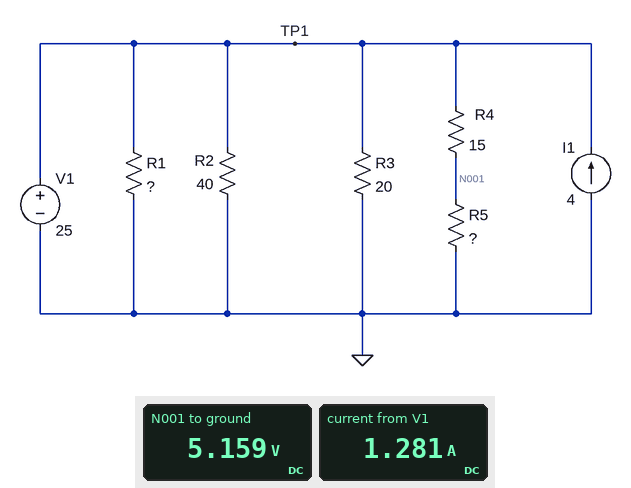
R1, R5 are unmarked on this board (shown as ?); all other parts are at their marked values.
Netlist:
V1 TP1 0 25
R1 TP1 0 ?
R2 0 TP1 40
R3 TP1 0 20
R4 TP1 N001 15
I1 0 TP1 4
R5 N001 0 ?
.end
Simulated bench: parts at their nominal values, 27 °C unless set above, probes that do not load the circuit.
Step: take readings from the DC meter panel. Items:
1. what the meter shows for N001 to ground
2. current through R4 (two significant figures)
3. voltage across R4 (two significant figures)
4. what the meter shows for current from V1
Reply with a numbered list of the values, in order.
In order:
1. 5.159 V
2. 1.3 A
3. 20 V
4. 1.281 A
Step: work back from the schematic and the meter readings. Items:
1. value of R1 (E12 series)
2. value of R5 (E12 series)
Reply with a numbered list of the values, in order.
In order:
1. 12 Ω
2. 3.9 Ω
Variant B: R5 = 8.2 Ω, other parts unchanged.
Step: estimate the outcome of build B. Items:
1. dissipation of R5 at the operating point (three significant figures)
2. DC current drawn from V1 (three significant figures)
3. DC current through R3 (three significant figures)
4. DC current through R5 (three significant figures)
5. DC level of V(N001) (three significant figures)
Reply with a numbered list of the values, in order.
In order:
1. 9.52 W
2. 1.04 A
3. 1.25 A
4. 1.08 A
5. 8.84 V
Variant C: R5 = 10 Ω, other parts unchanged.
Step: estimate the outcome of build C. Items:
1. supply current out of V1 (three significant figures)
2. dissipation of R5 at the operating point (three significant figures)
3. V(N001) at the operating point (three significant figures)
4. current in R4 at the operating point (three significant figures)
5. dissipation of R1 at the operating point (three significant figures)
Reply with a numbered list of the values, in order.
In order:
1. 958 mA
2. 10.0 W
3. 10.0 V
4. 1.00 A
5. 52.1 W
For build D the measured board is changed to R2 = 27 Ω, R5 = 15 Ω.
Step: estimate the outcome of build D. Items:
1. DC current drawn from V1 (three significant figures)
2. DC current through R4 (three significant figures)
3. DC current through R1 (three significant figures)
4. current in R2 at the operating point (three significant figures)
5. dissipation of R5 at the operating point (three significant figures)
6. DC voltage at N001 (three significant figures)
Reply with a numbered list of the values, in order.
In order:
1. 1.09 A
2. 833 mA
3. 2.08 A
4. 926 mA
5. 10.4 W
6. 12.5 V
